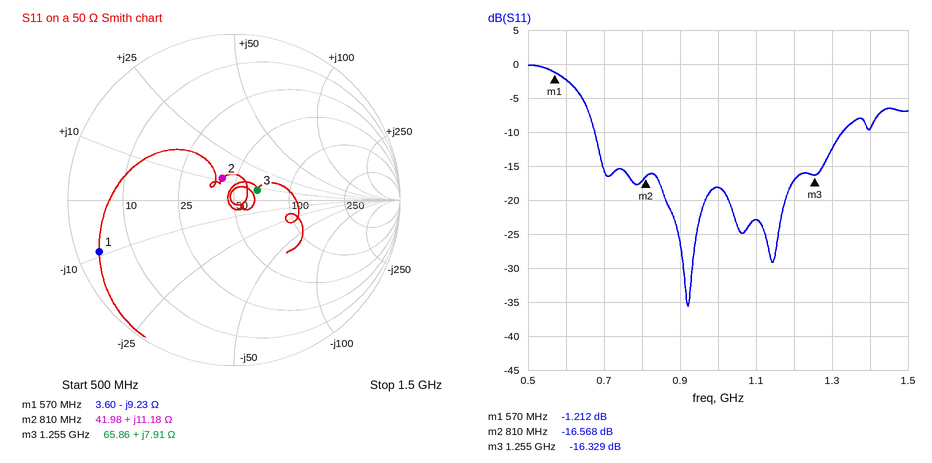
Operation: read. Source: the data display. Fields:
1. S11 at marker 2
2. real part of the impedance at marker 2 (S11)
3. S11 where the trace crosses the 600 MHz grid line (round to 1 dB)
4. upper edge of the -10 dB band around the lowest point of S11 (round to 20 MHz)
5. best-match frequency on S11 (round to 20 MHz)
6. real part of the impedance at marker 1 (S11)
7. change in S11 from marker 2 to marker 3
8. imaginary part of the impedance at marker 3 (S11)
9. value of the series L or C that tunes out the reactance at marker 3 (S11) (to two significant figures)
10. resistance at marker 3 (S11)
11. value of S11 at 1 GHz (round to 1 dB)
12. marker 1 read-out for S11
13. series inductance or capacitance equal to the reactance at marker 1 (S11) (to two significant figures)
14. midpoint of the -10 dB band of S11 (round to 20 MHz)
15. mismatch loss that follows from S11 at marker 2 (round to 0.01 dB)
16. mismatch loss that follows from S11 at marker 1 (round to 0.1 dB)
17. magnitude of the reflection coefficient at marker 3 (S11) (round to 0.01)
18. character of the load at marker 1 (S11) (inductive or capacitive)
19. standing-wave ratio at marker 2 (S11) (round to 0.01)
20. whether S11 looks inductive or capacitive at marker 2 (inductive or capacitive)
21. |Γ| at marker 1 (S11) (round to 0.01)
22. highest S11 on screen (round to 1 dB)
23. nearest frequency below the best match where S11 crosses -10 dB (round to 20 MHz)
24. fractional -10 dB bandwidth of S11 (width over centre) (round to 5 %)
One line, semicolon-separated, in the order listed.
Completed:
-16.568 dB; 41.98 Ω; -2 dB; 1.32 GHz; 920 MHz; 3.60 Ω; 0.239 dB; +7.91 Ω; 16 pF; 65.86 Ω; -18 dB; -1.212 dB; 30 pF; 1.00 GHz; 0.10 dB; 6.1 dB; 0.15; capacitive; 1.35; inductive; 0.87; 0 dB; 680 MHz; 65 %
